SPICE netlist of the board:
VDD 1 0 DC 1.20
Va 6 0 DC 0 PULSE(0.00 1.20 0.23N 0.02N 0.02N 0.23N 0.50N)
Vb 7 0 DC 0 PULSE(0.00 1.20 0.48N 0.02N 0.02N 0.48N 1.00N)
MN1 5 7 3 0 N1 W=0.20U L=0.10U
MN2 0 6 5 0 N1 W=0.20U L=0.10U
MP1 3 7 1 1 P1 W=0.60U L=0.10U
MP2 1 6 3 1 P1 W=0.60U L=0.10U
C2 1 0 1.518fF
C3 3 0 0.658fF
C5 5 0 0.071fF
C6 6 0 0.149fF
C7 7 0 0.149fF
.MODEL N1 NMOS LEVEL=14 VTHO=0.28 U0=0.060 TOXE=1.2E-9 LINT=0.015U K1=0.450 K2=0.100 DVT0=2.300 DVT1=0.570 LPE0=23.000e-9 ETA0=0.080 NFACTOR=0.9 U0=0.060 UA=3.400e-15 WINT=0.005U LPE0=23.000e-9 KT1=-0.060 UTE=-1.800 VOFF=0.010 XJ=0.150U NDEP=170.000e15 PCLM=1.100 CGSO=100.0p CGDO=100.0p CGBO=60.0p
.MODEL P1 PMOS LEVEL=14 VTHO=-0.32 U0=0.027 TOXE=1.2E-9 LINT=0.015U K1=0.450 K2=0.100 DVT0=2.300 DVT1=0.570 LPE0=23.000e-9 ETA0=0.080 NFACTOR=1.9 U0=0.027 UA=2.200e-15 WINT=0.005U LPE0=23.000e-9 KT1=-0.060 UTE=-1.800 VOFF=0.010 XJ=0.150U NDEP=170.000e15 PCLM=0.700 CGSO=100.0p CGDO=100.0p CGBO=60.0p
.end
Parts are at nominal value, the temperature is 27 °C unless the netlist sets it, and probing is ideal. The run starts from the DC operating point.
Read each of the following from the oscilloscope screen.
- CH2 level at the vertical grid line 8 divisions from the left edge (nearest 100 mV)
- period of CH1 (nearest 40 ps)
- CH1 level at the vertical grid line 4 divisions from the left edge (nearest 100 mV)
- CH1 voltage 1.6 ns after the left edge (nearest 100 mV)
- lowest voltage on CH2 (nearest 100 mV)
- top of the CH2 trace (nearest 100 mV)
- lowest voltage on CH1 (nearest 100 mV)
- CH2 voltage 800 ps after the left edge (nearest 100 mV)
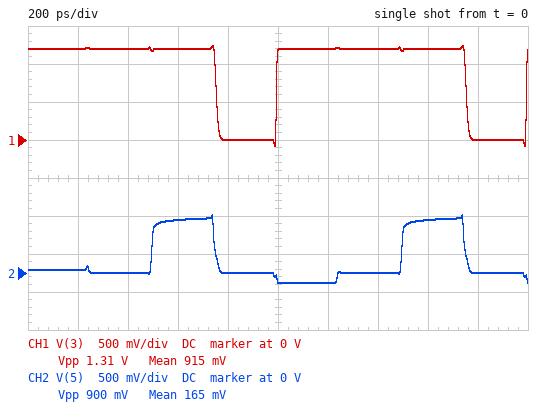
700 mV
1.00 ns
0 V
1.2 V
-100 mV
800 mV
-100 mV
0 V
